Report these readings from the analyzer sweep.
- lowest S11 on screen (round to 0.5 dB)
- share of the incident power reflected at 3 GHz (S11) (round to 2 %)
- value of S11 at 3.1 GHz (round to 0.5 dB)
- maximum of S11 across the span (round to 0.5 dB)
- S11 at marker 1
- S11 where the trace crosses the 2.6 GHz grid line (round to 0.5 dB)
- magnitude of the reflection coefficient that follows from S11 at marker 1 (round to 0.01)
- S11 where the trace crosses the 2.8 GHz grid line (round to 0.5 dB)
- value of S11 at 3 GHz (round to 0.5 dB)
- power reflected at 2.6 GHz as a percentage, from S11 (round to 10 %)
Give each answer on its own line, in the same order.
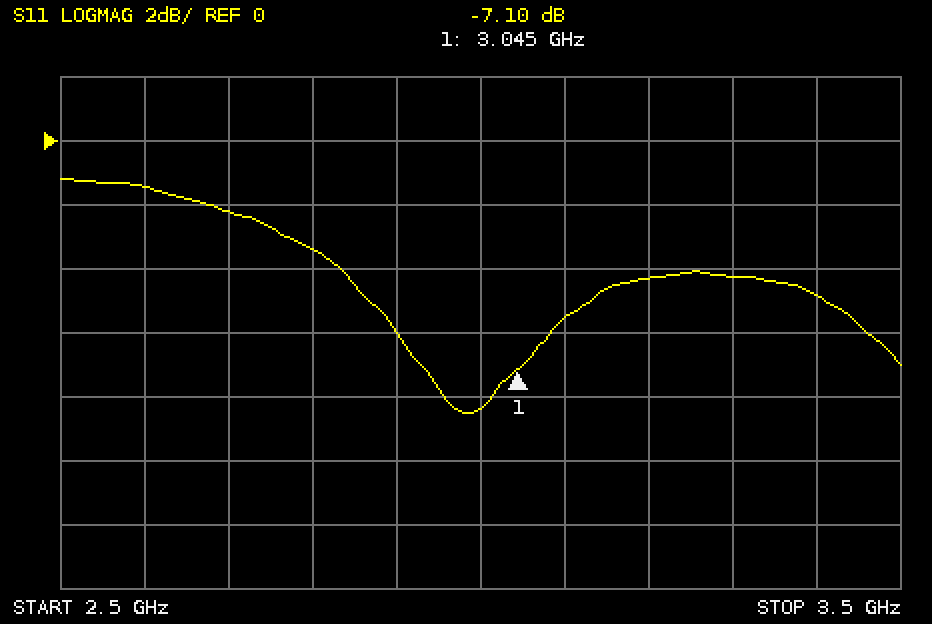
-8.5 dB
14 %
-5.5 dB
-1.0 dB
-7.10 dB
-1.5 dB
0.44
-3.5 dB
-8.5 dB
70 %
